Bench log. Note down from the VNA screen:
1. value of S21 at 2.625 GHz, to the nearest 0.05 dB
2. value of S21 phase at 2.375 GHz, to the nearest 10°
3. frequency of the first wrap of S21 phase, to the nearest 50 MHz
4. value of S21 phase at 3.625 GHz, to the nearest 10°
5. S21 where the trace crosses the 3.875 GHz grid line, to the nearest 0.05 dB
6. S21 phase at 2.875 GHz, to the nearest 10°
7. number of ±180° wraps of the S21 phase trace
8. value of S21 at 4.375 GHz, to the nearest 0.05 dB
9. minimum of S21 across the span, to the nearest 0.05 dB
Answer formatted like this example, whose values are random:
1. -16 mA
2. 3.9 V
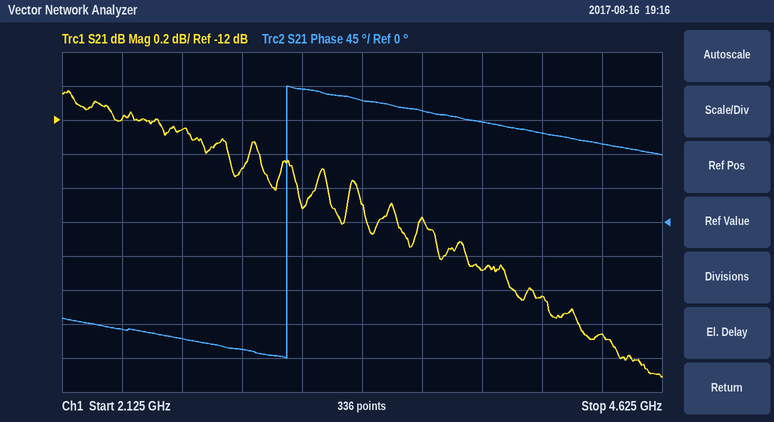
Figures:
1. -12.05 dB
2. -140°
3. 3.05 GHz
4. 150°
5. -12.90 dB
6. -170°
7. 1
8. -13.25 dB
9. -13.50 dB
